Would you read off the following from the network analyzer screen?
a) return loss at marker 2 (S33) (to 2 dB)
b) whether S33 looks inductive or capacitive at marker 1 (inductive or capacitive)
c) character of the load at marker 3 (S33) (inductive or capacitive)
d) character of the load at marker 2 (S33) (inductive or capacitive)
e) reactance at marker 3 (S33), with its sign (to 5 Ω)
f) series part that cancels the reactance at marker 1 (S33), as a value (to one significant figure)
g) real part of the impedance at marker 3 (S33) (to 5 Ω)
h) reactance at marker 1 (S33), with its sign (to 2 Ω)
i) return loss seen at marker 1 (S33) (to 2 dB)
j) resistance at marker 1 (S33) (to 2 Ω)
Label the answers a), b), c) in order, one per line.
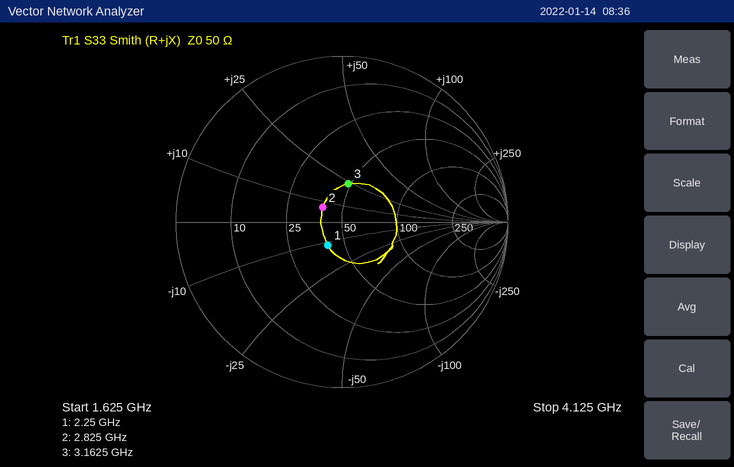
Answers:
a) 16 dB
b) capacitive
c) inductive
d) inductive
e) +25 Ω
f) 800 pH
g) 50 Ω
h) -12 Ω
i) 16 dB
j) 40 Ω
